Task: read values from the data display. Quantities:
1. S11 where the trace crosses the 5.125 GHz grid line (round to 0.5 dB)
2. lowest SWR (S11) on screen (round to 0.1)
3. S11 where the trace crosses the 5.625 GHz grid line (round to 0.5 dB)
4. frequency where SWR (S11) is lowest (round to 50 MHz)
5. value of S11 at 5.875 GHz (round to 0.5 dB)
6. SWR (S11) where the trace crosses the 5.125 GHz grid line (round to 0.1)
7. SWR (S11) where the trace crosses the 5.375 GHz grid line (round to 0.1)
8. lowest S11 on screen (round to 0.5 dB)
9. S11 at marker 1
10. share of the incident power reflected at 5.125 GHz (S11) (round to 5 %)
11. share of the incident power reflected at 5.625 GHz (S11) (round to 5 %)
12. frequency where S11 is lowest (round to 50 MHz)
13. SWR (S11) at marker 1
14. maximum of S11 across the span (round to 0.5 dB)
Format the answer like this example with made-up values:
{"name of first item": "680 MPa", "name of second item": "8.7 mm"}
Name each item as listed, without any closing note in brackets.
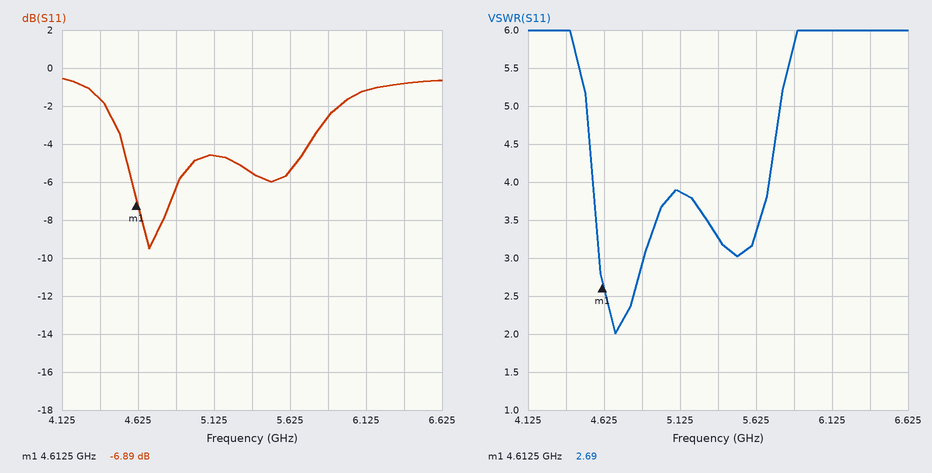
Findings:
{"S11 where the trace crosses the 5.125 GHz grid line": "-4.5 dB", "lowest SWR (S11) on screen": "2.0", "S11 where the trace crosses the 5.625 GHz grid line": "-5.5 dB", "frequency where SWR (S11) is lowest": "4.70 GHz", "value of S11 at 5.875 GHz": "-2.5 dB", "SWR (S11) where the trace crosses the 5.125 GHz grid line": "3.9", "SWR (S11) where the trace crosses the 5.375 GHz grid line": "3.3", "lowest S11 on screen": "-9.5 dB", "S11 at marker 1": "-6.89 dB", "share of the incident power reflected at 5.125 GHz (S11)": "35 %", "share of the incident power reflected at 5.625 GHz (S11)": "30 %", "frequency where S11 is lowest": "4.70 GHz", "SWR (S11) at marker 1": "2.69", "maximum of S11 across the span": "-0.5 dB"}
